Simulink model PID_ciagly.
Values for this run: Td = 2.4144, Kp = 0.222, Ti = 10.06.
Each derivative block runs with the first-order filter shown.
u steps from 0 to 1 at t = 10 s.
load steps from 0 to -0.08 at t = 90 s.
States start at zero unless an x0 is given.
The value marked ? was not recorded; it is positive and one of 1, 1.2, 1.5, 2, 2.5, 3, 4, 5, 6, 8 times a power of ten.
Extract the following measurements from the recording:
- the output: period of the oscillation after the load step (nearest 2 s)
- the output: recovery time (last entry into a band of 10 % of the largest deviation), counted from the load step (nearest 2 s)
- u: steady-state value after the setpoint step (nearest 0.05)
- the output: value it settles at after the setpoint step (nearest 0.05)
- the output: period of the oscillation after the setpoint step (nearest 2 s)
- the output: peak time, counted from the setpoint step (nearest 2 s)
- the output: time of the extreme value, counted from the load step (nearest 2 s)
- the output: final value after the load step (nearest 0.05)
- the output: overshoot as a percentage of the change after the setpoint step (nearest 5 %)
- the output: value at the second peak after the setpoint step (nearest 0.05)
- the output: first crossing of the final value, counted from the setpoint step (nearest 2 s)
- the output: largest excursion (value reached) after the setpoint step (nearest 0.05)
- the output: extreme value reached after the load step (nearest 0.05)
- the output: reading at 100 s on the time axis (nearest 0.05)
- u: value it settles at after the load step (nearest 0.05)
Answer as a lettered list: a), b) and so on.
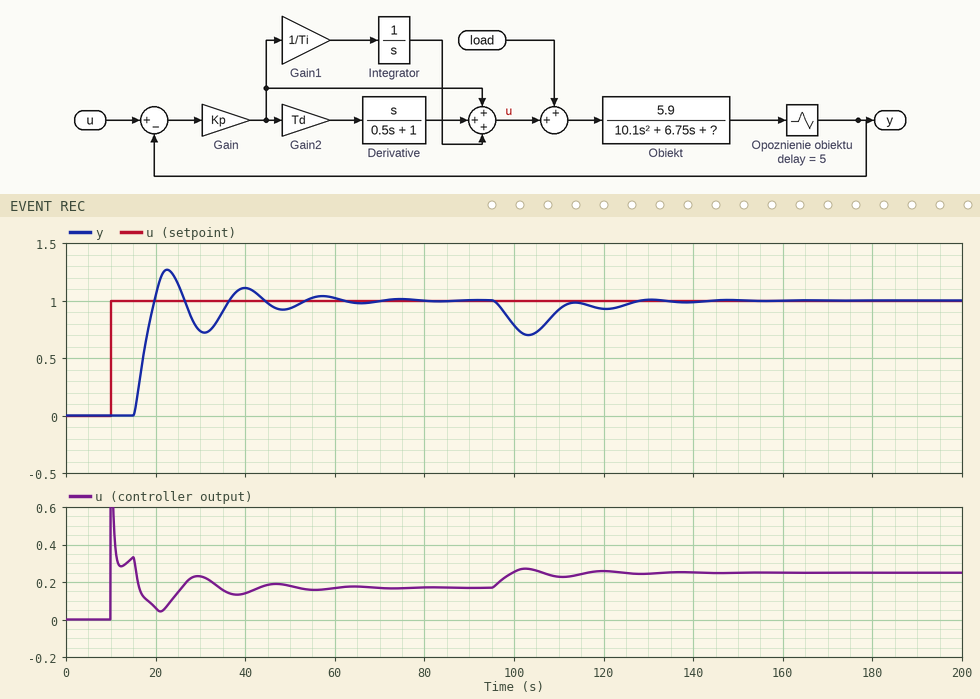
a) 18 s
b) 36 s
c) 0.15
d) 1.00
e) 18 s
f) 12 s
g) 14 s
h) 1.00
i) 25 %
j) 1.10
k) 10 s
l) 1.25
m) 0.70
n) 0.80
o) 0.25
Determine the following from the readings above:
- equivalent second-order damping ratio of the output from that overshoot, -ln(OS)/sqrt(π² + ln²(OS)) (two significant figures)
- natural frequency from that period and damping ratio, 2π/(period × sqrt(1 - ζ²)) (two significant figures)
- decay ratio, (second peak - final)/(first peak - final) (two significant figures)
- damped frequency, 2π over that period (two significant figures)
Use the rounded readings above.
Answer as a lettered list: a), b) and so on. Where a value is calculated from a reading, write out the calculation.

a) ln(0.25) = -1.386; 1.386 / sqrt(9.870 + 1.922) = 0.40
b) 2π / (18 × sqrt(1 - 0.4²)) = 0.38 rad/s
c) (1.1 - 1) / (1.25 - 1) = 0.40
d) 2π / 18 = 0.35 rad/s
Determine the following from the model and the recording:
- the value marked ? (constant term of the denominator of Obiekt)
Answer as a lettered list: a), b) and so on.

a) 1
